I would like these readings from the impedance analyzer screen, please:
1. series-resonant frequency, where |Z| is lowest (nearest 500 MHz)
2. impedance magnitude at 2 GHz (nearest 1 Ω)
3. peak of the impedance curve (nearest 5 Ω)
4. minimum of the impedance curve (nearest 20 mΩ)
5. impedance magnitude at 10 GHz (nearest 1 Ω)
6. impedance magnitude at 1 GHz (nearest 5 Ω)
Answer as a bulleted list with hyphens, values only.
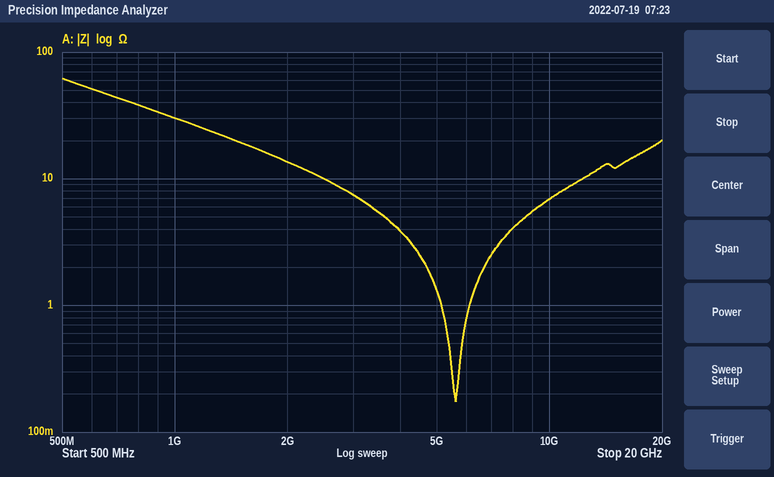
- 5.5 GHz
- 14 Ω
- 60 Ω
- 180 mΩ
- 7 Ω
- 30 Ω
